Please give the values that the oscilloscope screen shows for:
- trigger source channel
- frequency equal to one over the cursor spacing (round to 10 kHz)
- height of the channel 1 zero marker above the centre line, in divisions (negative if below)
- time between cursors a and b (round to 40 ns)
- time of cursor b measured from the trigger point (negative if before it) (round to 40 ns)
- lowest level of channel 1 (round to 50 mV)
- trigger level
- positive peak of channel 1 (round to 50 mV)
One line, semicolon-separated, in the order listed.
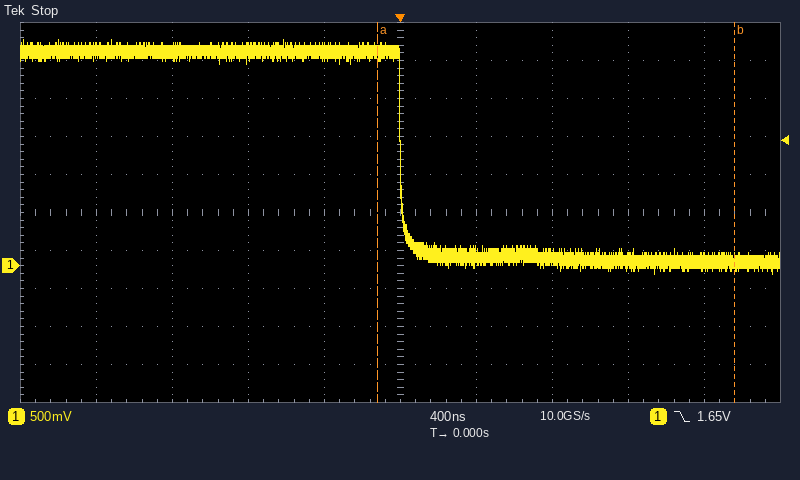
channel 1; 530 kHz; -1.4 div; 1.88 µs; +1.76 µs; -100 mV; 1.65 V; 3.00 V
